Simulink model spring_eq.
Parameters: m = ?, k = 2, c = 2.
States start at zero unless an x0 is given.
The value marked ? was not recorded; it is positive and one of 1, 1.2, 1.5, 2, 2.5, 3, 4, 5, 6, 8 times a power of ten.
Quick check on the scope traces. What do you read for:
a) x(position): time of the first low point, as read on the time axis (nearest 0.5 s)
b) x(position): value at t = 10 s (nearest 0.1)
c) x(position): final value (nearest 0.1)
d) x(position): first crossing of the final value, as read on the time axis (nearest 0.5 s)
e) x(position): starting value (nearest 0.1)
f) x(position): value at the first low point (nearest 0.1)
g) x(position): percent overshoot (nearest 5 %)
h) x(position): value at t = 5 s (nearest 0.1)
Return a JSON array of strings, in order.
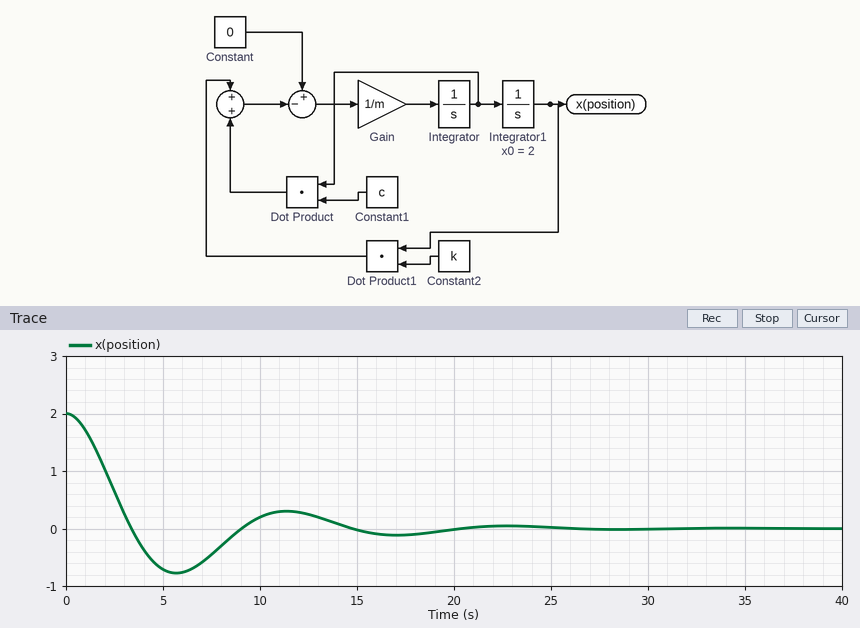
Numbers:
["5.5 s", "0.2", "0.0", "3.5 s", "2.0", "-0.8", "40 %", "-0.7"]
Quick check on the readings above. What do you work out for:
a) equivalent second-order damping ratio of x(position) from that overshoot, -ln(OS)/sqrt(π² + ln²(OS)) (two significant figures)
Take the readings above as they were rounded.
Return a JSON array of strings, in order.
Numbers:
["0.28"]
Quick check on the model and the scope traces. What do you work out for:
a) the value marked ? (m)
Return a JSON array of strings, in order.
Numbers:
["6"]
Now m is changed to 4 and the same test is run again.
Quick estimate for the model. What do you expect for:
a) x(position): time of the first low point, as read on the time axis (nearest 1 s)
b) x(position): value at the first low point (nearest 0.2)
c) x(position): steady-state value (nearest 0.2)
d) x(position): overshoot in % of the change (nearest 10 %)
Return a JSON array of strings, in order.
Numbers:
["5 s", "-0.6", "0.0", "30 %"]
